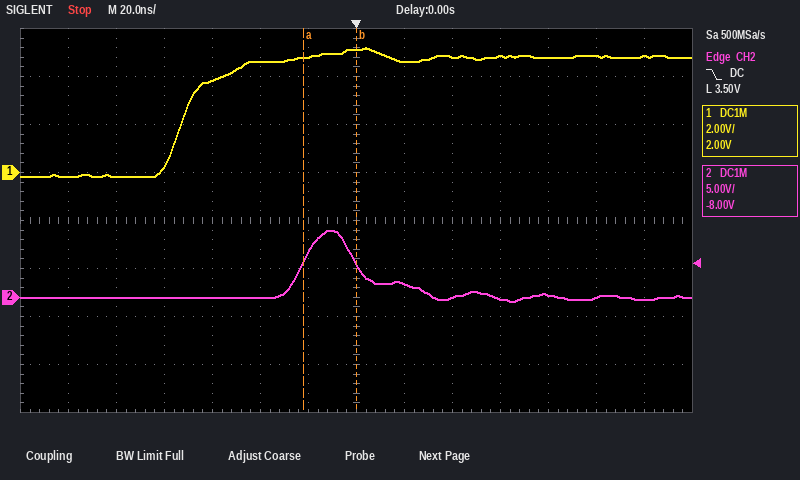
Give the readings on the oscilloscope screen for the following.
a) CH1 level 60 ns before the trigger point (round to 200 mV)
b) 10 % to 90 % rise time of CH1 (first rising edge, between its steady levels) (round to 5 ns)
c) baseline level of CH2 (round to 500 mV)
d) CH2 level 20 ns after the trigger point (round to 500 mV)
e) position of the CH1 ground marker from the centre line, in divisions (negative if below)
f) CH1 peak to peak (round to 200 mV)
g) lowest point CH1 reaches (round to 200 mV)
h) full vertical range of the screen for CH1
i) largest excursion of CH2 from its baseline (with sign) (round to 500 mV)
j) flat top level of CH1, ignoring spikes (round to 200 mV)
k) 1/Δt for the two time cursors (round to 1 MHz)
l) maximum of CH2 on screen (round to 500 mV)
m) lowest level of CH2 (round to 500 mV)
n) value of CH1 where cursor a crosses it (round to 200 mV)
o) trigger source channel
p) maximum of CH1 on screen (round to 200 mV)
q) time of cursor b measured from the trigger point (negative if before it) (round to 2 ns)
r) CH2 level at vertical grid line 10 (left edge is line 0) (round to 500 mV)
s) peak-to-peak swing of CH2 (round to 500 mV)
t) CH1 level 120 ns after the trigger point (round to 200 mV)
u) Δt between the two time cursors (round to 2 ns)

3.8 V
30 ns
0.0 V
1.5 V
+1.0 div
5.4 V
-200 mV
16 V
+7.0 V
4.8 V
45 MHz
7.0 V
-500 mV
4.8 V
CH2
5.2 V
0 ns
0.0 V
7.5 V
4.8 V
22 ns
